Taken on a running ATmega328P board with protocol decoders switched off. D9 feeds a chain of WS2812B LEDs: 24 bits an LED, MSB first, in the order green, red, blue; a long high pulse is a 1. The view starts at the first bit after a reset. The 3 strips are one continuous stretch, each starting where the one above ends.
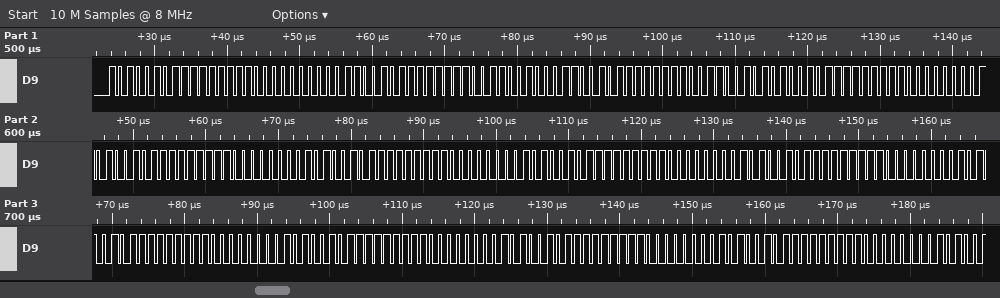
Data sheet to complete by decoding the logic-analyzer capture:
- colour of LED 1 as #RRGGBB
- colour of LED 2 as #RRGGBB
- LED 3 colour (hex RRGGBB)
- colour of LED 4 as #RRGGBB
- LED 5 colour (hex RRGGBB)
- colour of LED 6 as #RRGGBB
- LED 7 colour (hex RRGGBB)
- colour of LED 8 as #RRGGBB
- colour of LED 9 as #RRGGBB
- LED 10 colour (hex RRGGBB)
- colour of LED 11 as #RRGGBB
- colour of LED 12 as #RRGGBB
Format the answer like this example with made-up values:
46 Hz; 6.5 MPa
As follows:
#FFA500; #FF3232; #FF3232; #FFA500; #FFA500; #FFA500; #FFA500; #FFA500; #FFA500; #FFA500; #FFA500; #FFA500
